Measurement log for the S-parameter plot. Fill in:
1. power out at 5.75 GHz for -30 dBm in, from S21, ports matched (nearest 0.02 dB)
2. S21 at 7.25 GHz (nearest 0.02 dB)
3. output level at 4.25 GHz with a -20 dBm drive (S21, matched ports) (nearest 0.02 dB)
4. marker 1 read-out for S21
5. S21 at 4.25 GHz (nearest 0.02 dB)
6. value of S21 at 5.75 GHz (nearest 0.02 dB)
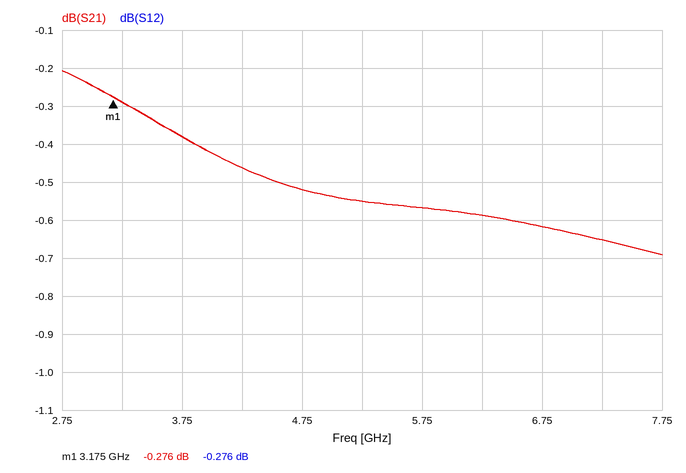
-30.56 dBm
-0.66 dB
-20.46 dBm
-0.276 dB
-0.46 dB
-0.56 dB
